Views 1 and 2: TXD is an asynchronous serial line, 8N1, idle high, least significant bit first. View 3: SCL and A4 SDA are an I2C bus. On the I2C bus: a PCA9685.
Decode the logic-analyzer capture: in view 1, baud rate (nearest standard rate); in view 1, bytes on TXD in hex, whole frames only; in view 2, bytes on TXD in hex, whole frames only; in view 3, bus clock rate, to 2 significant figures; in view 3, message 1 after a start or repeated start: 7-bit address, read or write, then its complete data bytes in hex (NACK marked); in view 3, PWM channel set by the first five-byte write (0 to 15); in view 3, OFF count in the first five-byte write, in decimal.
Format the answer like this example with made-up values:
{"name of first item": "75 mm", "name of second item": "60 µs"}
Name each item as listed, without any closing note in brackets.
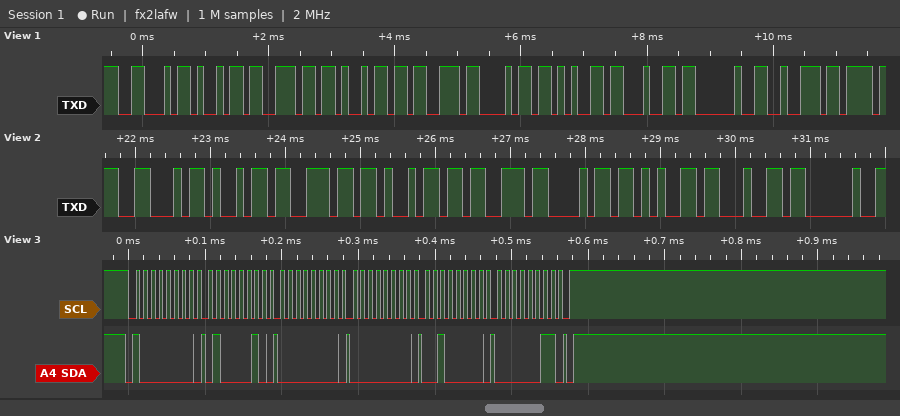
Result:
{"in view 1, baud rate": "9600 baud", "in view 1, bytes on TXD in hex, whole frames only": "0x46 0x69 0x6E 0x69 0x73 0x68 0x65 0x64 0x20 0x72", "in view 2, bytes on TXD in hex, whole frames only": "46 69 6E 69 73 68 65 64 20", "in view 3, bus clock rate, to 2 significant figures": "100 kHz", "in view 3, message 1 after a start or repeated start: 7-bit address, read or write, then its complete data bytes in hex": "0x40 write: 42 00 00 20 03", "in view 3, PWM channel set by the first five-byte write": "15", "in view 3, OFF count in the first five-byte write, in decimal": "800"}
